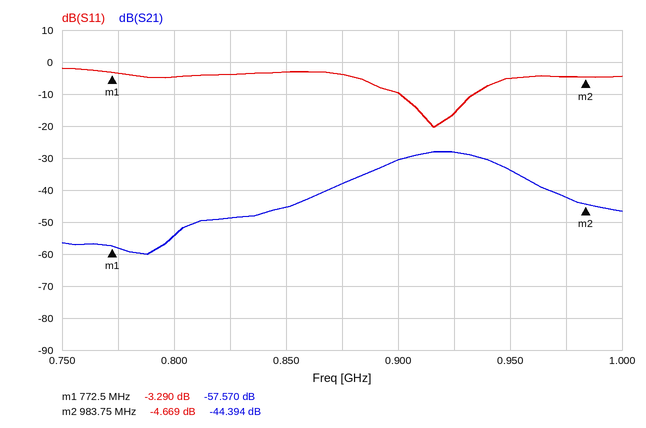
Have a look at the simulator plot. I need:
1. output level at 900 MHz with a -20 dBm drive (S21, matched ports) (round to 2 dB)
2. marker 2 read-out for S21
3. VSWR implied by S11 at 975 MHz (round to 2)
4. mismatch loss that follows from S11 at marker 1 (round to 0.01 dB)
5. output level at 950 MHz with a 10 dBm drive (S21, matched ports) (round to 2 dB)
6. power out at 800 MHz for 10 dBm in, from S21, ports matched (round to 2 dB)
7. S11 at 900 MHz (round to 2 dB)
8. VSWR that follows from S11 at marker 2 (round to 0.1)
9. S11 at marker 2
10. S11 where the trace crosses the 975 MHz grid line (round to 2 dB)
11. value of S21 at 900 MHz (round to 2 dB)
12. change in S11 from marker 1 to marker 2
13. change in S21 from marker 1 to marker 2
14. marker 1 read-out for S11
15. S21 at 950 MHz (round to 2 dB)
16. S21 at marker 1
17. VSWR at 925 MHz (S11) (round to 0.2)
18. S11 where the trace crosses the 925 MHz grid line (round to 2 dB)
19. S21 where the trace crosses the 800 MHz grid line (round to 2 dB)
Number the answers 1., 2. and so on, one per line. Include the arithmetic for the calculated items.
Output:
1. -20 dBm + (-30 dB) = -50 dBm
2. -44.394 dB
3. |Γ| = 10^(-4/20) = 0.6310; VSWR = (1 + 0.6310)/(1 − 0.6310) ≈ 4
4. −10 log10(1 − 10^(-3.29/10)) ≈ 2.75 dB
5. 10 dBm + (-34 dB) = -24 dBm
6. 10 dBm + (-54 dB) = -44 dBm
7. -10 dB
8. (1 + 0.5842)/(1 − 0.5842) ≈ 3.8
9. -4.669 dB
10. -4 dB
11. -30 dB
12. -4.669 − (-3.29) = -1.379 dB
13. -44.394 − (-57.57) = 13.176 dB
14. -3.290 dB
15. -34 dB
16. -57.570 dB
17. |Γ| = 10^(-16/20) = 0.1585; VSWR = (1 + 0.1585)/(1 − 0.1585) ≈ 1.4
18. -16 dB
19. -54 dB
